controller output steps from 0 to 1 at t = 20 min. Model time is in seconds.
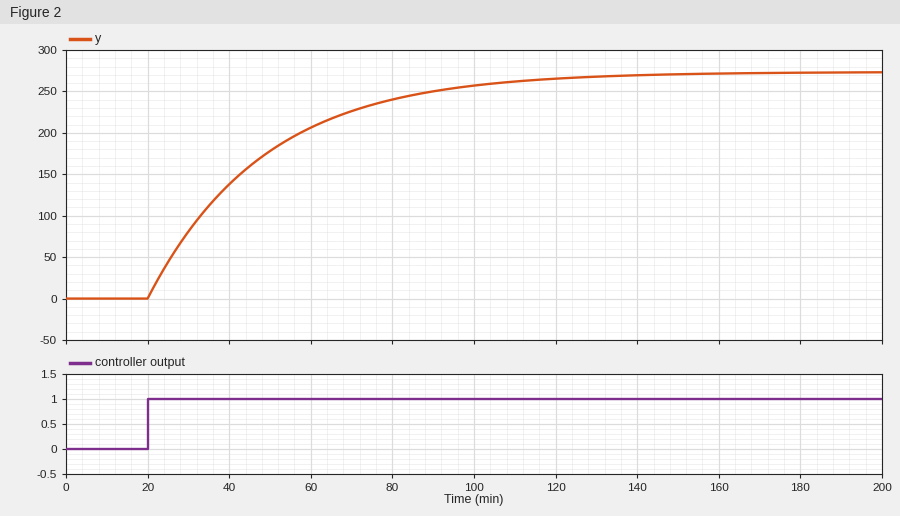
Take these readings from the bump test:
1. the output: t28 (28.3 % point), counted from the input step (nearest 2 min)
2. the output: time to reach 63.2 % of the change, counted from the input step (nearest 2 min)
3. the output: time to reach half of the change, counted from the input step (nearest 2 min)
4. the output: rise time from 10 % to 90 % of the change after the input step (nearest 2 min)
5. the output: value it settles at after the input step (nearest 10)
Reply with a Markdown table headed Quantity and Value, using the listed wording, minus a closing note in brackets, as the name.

| Quantity | Value |
|---|---|
| the output: t28 (28.3 % point), counted from the input step | 10 min |
| the output: time to reach 63.2 % of the change, counted from the input step | 28 min |
| the output: time to reach half of the change, counted from the input step | 20 min |
| the output: rise time from 10 % to 90 % of the change after the input step | 62 min |
| the output: value it settles at after the input step | 270 |
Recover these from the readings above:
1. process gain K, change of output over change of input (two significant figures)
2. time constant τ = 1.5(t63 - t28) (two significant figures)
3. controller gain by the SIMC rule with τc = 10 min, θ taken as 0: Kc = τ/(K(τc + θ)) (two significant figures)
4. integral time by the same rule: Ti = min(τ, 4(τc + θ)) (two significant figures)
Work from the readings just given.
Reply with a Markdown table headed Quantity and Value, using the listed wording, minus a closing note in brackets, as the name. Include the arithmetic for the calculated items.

| Quantity | Value |
|---|---|
| process gain K, change of output over change of input | (270 - 0) / 1 = 270 |
| time constant τ = 1.5(t63 - t28) | 1.5 × (28 - 10) = 27 min |
| controller gain by the SIMC rule with τc = 10 min, θ taken as 0: Kc = τ/(K(τc + θ)) | 27 / (270 × (10 + 0)) = 0.010 |
| integral time by the same rule: Ti = min(τ, 4(τc + θ)) | min(27, 4 × (10 + 0)) = 27 min |
